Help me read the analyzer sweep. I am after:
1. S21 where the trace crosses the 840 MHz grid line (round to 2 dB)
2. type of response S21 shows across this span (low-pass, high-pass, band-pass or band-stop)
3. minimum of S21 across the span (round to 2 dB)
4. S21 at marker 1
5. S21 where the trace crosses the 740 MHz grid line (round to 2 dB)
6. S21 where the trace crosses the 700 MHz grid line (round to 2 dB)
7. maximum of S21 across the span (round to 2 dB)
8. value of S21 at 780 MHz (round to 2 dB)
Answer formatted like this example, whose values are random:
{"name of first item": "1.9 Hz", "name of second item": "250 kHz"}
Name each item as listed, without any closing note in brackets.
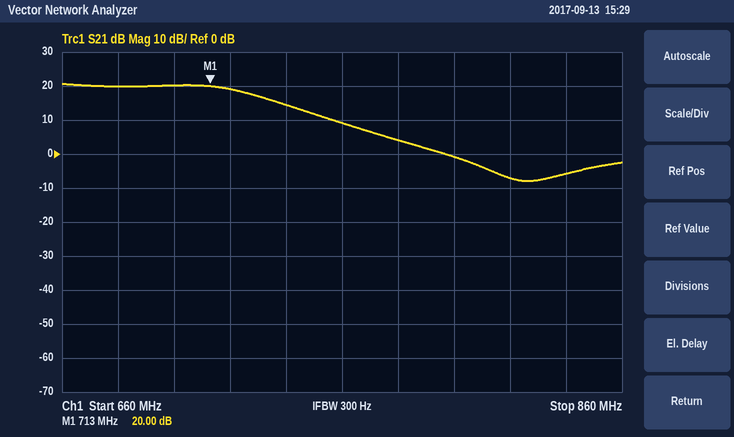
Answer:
{"S21 where the trace crosses the 840 MHz grid line": "-6 dB", "type of response S21 shows across this span": "low-pass", "minimum of S21 across the span": "-8 dB", "S21 at marker 1": "20.00 dB", "S21 where the trace crosses the 740 MHz grid line": "14 dB", "S21 where the trace crosses the 700 MHz grid line": "20 dB", "maximum of S21 across the span": "20 dB", "value of S21 at 780 MHz": "4 dB"}
